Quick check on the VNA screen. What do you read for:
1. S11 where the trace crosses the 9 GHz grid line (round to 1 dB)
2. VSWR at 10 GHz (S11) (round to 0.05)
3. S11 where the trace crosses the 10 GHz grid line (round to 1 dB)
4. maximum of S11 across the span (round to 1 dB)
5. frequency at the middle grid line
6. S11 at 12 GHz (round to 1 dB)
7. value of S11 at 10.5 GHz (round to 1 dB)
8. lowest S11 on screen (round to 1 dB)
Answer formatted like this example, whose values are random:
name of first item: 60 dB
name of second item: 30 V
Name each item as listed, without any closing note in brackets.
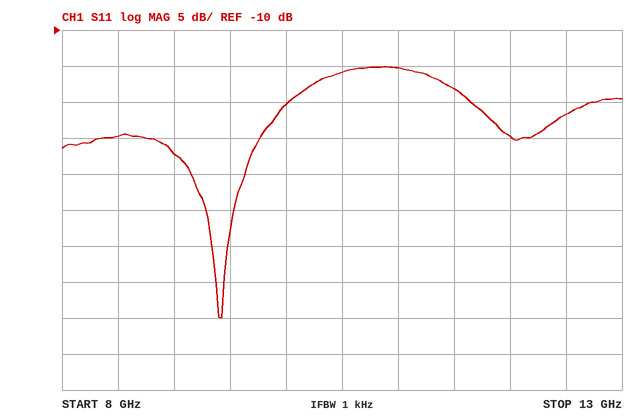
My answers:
S11 where the trace crosses the 9 GHz grid line: -27 dB
VSWR at 10 GHz (S11): 1.20
S11 where the trace crosses the 10 GHz grid line: -20 dB
maximum of S11 across the span: -15 dB
frequency at the middle grid line: 10.5 GHz
S11 at 12 GHz: -25 dB
value of S11 at 10.5 GHz: -16 dB
lowest S11 on screen: -50 dB
